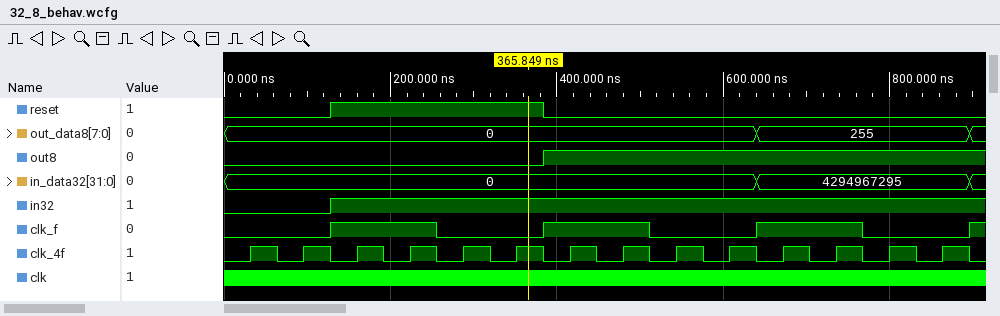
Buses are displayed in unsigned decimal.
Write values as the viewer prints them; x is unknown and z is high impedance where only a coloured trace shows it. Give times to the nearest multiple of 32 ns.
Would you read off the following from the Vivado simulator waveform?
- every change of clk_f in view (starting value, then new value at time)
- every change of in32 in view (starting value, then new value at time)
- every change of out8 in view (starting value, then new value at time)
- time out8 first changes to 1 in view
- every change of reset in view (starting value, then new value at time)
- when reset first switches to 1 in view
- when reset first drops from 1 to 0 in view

0, 1 at 128 ns, 0 at 256 ns, 1 at 384 ns, 0 at 512 ns, 1 at 640 ns, 0 at 768 ns, 1 at 896 ns
0, 1 at 128 ns
0, 1 at 384 ns
384 ns
0, 1 at 128 ns, 0 at 384 ns
128 ns
384 ns
